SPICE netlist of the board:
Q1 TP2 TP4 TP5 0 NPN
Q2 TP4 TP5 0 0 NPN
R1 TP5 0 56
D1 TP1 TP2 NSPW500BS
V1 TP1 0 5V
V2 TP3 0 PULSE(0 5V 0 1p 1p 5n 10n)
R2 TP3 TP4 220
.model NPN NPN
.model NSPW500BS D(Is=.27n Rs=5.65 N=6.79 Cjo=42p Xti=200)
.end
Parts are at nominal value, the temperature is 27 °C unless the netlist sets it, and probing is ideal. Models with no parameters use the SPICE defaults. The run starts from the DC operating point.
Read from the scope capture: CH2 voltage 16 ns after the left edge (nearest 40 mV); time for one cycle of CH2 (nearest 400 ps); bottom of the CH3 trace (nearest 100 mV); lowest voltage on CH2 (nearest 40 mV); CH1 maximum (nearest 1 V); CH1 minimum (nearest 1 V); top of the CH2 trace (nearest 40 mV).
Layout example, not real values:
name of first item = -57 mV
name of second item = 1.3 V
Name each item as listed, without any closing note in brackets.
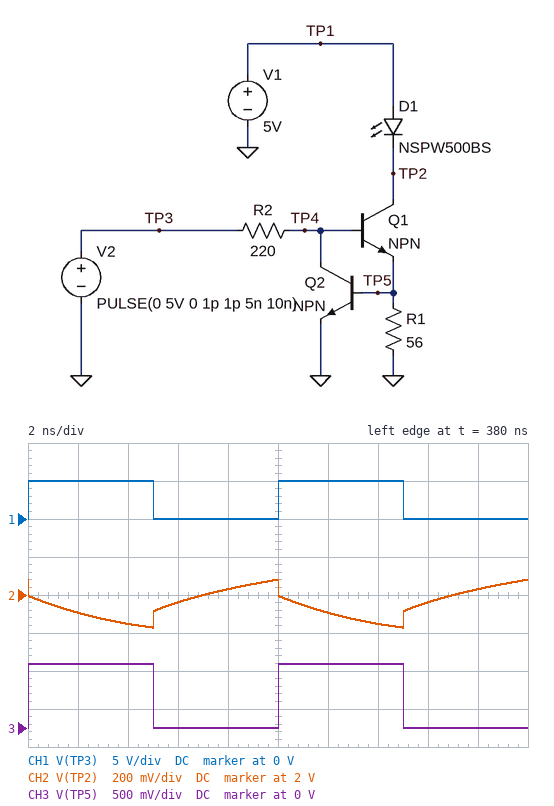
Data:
CH2 voltage 16 ns after the left edge = 1.96 V
time for one cycle of CH2 = 10.0 ns
bottom of the CH3 trace = 0 V
lowest voltage on CH2 = 1.84 V
CH1 maximum = 5 V
CH1 minimum = 0 V
top of the CH2 trace = 2.08 V
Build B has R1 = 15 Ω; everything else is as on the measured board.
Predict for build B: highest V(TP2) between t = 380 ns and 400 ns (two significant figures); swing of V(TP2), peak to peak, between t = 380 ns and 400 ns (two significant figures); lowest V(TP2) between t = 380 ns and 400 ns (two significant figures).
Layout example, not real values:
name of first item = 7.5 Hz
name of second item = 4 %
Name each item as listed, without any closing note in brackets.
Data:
highest V(TP2) between t = 380 ns and 400 ns = 2.0 V
swing of V(TP2), peak to peak, between t = 380 ns and 400 ns = 690 mV
lowest V(TP2) between t = 380 ns and 400 ns = 1.3 V
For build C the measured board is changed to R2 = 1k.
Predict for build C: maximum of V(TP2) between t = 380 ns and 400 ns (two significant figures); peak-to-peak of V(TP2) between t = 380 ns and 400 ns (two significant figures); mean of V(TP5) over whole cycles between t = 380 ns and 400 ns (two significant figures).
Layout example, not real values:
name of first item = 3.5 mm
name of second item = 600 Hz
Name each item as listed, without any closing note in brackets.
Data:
maximum of V(TP2) between t = 380 ns and 400 ns = 2.1 V
peak-to-peak of V(TP2) between t = 380 ns and 400 ns = 240 mV
mean of V(TP5) over whole cycles between t = 380 ns and 400 ns = 400 mV
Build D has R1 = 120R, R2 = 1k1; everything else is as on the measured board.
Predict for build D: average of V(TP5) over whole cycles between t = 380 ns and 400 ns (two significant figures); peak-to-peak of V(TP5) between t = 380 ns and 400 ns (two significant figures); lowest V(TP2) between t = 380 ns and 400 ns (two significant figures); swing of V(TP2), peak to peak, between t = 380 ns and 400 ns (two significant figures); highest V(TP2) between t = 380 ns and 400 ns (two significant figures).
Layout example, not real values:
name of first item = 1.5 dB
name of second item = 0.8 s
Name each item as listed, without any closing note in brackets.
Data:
average of V(TP5) over whole cycles between t = 380 ns and 400 ns = 400 mV
peak-to-peak of V(TP5) between t = 380 ns and 400 ns = 800 mV
lowest V(TP2) between t = 380 ns and 400 ns = 2.1 V
swing of V(TP2), peak to peak, between t = 380 ns and 400 ns = 120 mV
highest V(TP2) between t = 380 ns and 400 ns = 2.2 V
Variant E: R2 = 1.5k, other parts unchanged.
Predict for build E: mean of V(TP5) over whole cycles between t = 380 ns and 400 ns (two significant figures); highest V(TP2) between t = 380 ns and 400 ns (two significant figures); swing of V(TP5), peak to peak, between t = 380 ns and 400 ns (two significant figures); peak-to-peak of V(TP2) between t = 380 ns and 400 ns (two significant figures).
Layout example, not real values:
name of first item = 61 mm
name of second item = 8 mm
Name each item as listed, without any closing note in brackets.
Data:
mean of V(TP5) over whole cycles between t = 380 ns and 400 ns = 400 mV
highest V(TP2) between t = 380 ns and 400 ns = 2.1 V
swing of V(TP5), peak to peak, between t = 380 ns and 400 ns = 790 mV
peak-to-peak of V(TP2) between t = 380 ns and 400 ns = 240 mV
